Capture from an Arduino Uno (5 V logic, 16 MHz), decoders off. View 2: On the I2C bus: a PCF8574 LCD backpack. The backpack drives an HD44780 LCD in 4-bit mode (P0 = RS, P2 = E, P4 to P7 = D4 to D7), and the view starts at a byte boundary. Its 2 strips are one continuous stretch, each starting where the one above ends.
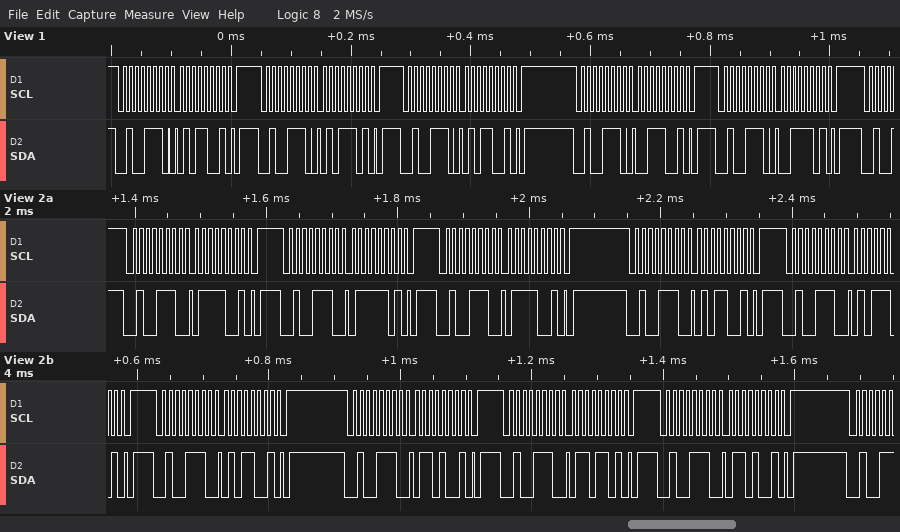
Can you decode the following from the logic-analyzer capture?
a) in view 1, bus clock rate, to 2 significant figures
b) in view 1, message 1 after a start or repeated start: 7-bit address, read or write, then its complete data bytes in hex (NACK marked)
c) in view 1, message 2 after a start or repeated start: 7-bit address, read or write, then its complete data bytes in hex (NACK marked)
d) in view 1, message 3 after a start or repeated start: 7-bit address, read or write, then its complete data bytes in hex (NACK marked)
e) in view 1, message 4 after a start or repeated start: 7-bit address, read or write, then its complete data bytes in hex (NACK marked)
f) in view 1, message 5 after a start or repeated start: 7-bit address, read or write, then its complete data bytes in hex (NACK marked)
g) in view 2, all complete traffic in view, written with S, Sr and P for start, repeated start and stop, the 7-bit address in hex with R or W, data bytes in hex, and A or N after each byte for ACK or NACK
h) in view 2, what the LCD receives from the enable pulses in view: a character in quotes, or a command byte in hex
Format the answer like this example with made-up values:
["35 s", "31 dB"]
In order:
["100 kHz", "0x27 write: 59", "0x27 write: 5D", "0x27 write: 59", "0x27 write: 39", "0x27 write: 3D", "S 27W A 79 A P S 27W A 7D A P S 27W A 79 A P S 27W A 59 A P S 27W A 5D A P S 27W A 59 A P S 27W A 69 A P S 27W A 6D A P S 27W A 69 A P", "'u'"]
